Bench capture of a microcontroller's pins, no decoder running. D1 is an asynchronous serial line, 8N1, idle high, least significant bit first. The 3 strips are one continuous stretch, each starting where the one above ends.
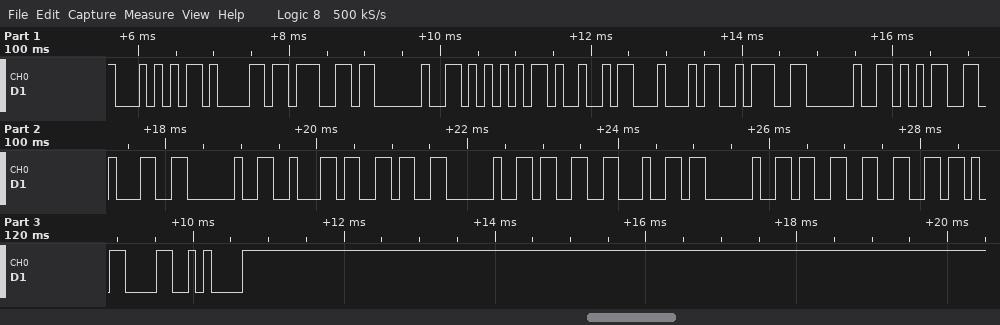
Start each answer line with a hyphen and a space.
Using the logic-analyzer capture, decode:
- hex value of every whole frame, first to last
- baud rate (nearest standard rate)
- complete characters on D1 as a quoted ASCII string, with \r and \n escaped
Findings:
- 54 61 67 20 55 49 44 3A 20 35 31 20 62 36 20 33 64 20 33 66 0D 0A
- 9600 baud
- "Tag UID: 51 b6 3d 3f\r\n"
